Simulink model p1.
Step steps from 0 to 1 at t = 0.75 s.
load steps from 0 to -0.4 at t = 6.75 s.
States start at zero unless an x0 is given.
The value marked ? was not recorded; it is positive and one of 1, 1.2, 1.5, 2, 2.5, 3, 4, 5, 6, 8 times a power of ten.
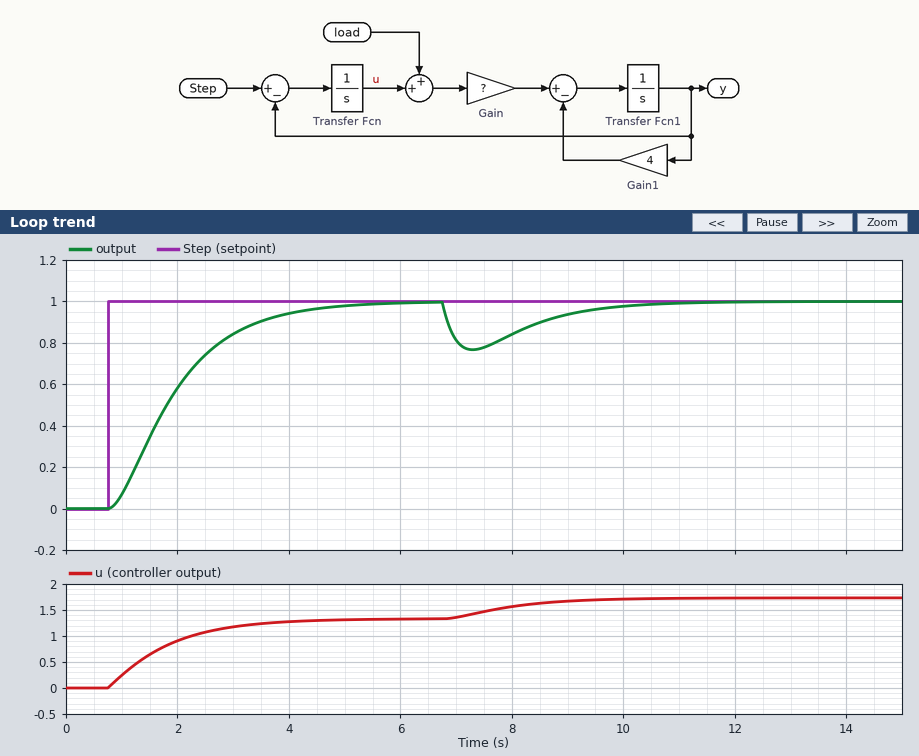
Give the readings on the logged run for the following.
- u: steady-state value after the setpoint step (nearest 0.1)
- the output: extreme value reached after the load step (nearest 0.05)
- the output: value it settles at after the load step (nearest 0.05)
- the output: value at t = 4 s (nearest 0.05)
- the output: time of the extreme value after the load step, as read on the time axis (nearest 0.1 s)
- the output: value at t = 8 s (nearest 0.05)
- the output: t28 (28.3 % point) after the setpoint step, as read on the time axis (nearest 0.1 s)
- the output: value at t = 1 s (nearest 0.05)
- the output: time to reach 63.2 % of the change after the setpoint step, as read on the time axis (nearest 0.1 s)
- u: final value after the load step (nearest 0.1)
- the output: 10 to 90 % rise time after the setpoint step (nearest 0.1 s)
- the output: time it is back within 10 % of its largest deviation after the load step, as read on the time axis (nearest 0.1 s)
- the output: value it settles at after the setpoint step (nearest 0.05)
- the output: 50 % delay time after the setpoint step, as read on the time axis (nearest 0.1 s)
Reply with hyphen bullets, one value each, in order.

- 1.3
- 0.75
- 1.00
- 0.95
- 7.3 s
- 0.85
- 1.4 s
- 0.05
- 2.1 s
- 1.7
- 2.4 s
- 10.0 s
- 1.00
- 1.8 s
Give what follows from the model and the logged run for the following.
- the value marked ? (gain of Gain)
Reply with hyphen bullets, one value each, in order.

- 3
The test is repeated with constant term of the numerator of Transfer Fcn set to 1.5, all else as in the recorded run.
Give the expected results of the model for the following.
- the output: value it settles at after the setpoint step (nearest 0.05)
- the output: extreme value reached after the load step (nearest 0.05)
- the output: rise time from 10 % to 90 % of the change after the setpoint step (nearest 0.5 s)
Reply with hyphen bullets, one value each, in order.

- 1.00
- 0.80
- 1.5 s
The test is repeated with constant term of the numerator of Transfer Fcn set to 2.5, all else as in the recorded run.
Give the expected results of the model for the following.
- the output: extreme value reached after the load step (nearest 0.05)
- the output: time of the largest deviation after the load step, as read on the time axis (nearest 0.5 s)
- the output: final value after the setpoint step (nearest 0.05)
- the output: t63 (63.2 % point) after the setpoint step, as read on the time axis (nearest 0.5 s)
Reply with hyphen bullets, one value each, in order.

- 0.80
- 7.0 s
- 1.00
- 1.5 s
